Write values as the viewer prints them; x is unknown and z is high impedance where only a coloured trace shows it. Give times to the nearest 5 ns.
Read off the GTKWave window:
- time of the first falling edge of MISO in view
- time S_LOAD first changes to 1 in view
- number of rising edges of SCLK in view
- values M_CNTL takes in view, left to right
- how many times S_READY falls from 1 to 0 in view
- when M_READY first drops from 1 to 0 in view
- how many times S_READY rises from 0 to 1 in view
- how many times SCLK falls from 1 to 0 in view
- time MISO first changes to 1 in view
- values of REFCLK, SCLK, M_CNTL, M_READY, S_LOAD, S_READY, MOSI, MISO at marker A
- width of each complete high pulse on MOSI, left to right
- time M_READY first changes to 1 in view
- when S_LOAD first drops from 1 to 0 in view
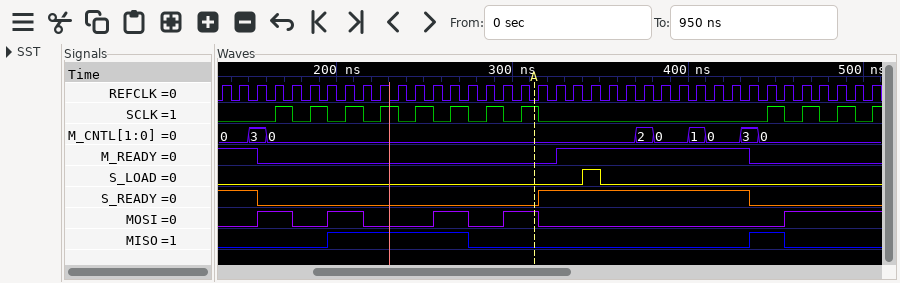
275 ns
340 ns
12
0, 3, 0, 2, 0, 1, 0, 3, 0
2
155 ns
1
11
195 ns
REFCLK=0, SCLK=1, M_CNTL=0, M_READY=0, S_LOAD=0, S_READY=0, MOSI=1, MISO=0
20 ns, 20 ns, 20 ns, 20 ns
325 ns
350 ns
